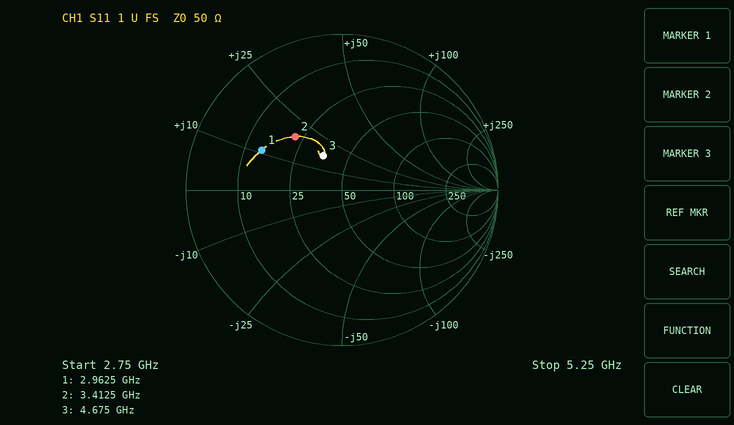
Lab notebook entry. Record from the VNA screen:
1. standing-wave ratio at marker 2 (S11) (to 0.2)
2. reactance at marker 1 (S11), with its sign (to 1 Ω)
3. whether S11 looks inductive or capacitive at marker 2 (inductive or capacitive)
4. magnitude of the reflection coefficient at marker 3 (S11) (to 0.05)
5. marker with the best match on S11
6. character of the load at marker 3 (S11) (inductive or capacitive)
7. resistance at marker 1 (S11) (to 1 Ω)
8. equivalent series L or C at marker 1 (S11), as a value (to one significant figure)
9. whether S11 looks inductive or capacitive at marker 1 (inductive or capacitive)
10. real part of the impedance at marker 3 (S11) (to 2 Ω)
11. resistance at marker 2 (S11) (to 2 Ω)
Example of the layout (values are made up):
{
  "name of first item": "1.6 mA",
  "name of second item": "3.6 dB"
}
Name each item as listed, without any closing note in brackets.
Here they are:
{
  "standing-wave ratio at marker 2 (S11)": "2.6",
  "reactance at marker 1 (S11), with its sign": "+11 Ω",
  "whether S11 looks inductive or capacitive at marker 2": "inductive",
  "magnitude of the reflection coefficient at marker 3 (S11)": "0.25",
  "marker with the best match on S11": "marker 3",
  "character of the load at marker 3 (S11)": "inductive",
  "resistance at marker 1 (S11)": "14 Ω",
  "equivalent series L or C at marker 1 (S11), as a value": "600 pH",
  "whether S11 looks inductive or capacitive at marker 1": "inductive",
  "real part of the impedance at marker 3 (S11)": "36 Ω",
  "resistance at marker 2 (S11)": "22 Ω"
}
